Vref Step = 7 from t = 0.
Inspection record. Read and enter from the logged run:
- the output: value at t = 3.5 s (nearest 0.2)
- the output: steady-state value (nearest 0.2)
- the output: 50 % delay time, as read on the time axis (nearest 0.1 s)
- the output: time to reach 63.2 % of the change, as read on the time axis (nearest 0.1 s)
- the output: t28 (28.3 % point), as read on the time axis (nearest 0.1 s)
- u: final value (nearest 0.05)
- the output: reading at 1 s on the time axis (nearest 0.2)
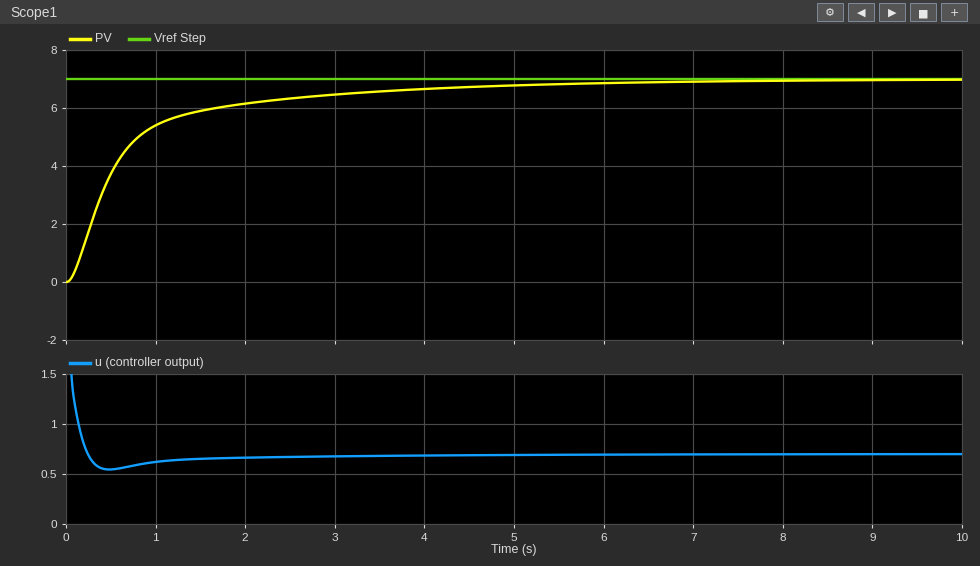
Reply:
6.6
7.0
0.5 s
0.6 s
0.3 s
0.70
5.4
